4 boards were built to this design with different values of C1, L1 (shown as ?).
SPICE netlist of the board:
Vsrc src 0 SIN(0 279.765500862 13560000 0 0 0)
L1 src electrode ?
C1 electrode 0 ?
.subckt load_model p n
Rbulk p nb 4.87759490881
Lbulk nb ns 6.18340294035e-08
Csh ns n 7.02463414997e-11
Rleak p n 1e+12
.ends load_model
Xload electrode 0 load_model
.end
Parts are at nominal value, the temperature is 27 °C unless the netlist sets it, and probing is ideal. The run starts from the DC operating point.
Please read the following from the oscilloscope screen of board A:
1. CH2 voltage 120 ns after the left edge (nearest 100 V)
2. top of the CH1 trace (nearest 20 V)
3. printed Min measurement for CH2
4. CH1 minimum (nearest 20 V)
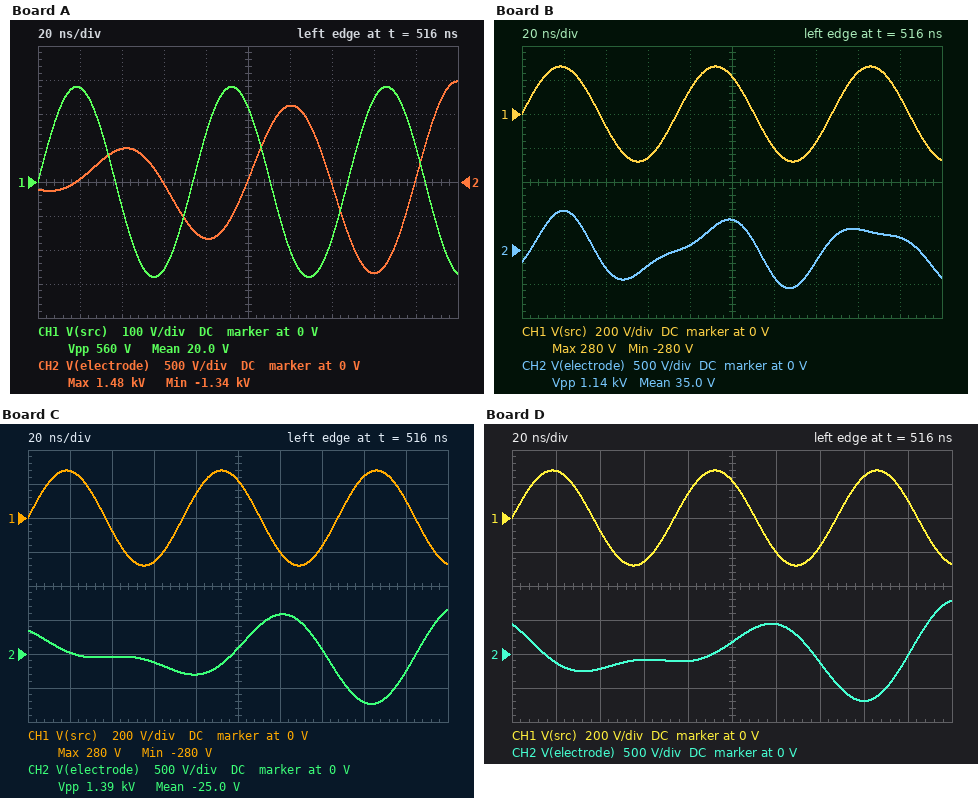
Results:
1.1 kV
280 V
-1.34 kV
-280 V
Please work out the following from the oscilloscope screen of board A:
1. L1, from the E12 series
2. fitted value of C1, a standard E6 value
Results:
470 nH
330 pF
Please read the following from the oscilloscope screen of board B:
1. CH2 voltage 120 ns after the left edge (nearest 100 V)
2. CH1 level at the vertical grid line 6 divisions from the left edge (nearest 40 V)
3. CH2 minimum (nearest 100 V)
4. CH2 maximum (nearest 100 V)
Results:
-400 V
-200 V
-600 V
600 V
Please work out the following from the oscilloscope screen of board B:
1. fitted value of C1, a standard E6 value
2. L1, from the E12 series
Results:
470 pF
82 nH
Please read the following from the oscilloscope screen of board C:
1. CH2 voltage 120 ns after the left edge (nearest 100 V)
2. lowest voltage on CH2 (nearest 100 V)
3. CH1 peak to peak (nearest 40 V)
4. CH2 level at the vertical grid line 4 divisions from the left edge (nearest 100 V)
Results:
600 V
-700 V
560 V
-300 V
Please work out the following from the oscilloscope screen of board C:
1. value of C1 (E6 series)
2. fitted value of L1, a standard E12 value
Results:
470 pF
470 nH
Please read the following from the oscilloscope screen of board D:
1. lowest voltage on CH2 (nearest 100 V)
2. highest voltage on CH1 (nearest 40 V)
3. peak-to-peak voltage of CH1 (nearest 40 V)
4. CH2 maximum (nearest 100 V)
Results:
-700 V
280 V
560 V
800 V
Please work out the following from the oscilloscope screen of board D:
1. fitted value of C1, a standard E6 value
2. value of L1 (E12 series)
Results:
680 pF
330 nH
